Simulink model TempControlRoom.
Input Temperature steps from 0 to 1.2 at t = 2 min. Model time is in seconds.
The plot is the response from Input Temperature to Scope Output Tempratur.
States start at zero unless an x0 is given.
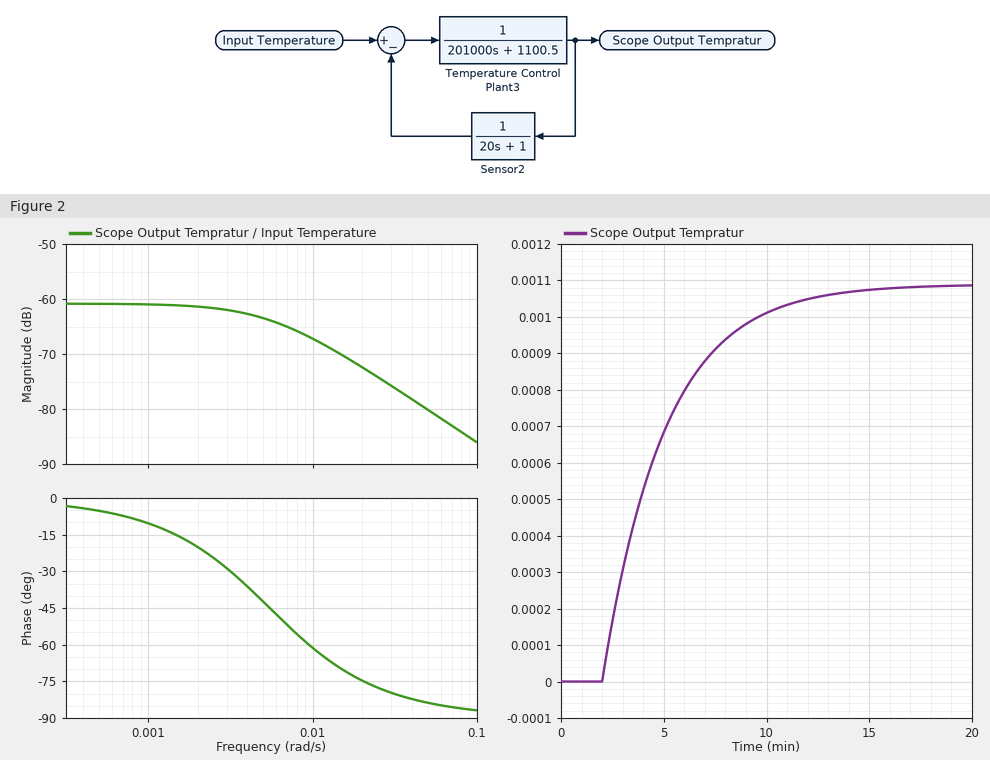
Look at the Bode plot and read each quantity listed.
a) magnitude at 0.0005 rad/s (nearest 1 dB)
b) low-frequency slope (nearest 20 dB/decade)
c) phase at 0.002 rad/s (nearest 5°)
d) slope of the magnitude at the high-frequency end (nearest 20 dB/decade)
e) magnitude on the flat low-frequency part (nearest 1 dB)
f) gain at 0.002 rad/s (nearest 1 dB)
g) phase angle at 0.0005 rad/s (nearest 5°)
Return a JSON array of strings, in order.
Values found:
["-61 dB", "0 dB/decade", "-20°", "-20 dB/decade", "-61 dB", "-61 dB", "-5°"]
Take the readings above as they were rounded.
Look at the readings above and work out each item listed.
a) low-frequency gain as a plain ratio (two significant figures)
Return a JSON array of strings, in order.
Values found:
["0.00089"]
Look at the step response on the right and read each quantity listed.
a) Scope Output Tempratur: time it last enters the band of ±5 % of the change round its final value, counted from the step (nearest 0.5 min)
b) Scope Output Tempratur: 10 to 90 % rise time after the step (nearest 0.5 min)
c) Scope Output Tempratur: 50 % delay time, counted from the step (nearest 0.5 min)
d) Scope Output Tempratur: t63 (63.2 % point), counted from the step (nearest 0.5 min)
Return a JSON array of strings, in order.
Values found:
["9.0 min", "6.5 min", "2.0 min", "3.0 min"]
